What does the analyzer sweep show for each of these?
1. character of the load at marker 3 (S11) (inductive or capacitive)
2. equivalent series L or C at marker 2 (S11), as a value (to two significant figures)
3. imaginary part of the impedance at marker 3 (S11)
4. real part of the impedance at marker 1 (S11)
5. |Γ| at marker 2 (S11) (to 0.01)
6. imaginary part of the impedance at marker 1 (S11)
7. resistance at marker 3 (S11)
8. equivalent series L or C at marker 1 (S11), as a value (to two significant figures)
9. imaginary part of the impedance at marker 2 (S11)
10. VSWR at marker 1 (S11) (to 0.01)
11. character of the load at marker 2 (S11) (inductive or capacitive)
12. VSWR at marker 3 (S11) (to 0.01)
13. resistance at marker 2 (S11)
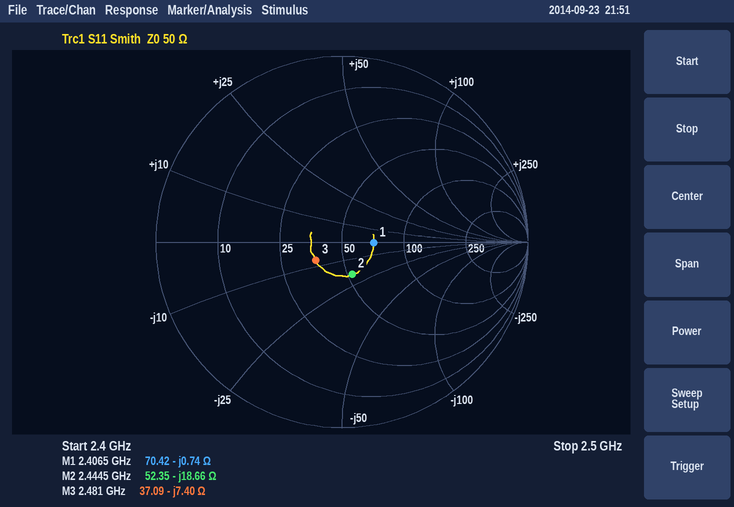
capacitive
3.5 pF
-7.40 Ω
70.42 Ω
0.18
-0.74 Ω
37.09 Ω
89 pF
-18.66 Ω
1.41
capacitive
1.41
52.35 Ω
